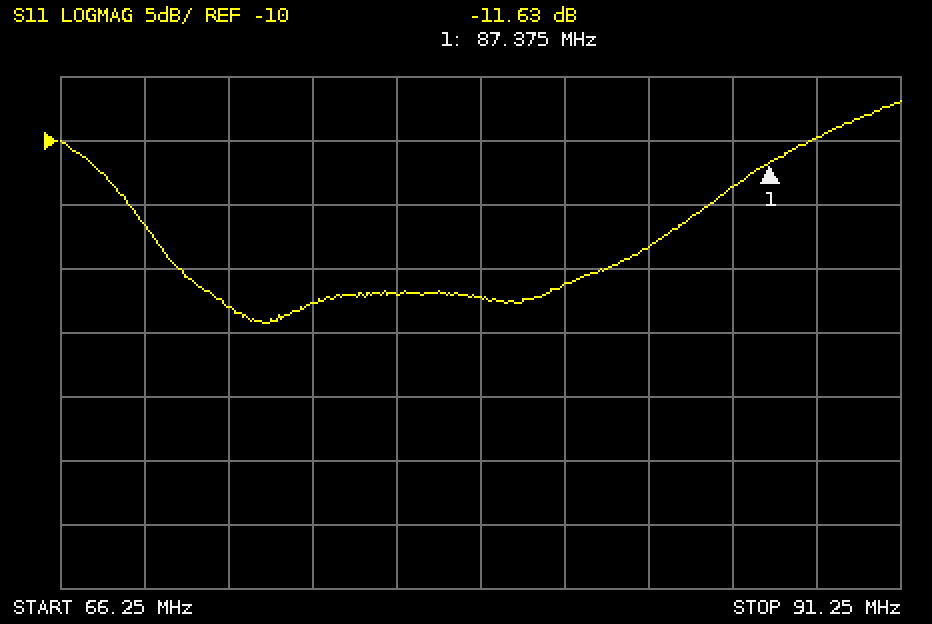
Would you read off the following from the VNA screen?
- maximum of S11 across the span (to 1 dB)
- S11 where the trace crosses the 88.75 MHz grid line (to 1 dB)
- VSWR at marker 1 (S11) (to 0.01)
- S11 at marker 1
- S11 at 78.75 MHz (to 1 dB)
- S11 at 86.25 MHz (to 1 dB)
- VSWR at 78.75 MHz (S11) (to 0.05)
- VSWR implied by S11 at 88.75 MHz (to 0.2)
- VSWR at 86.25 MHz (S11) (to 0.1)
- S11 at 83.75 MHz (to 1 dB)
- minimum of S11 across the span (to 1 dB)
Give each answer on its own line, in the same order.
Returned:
-7 dB
-10 dB
1.71
-11.63 dB
-22 dB
-14 dB
1.15
2.0
1.5
-18 dB
-24 dB
